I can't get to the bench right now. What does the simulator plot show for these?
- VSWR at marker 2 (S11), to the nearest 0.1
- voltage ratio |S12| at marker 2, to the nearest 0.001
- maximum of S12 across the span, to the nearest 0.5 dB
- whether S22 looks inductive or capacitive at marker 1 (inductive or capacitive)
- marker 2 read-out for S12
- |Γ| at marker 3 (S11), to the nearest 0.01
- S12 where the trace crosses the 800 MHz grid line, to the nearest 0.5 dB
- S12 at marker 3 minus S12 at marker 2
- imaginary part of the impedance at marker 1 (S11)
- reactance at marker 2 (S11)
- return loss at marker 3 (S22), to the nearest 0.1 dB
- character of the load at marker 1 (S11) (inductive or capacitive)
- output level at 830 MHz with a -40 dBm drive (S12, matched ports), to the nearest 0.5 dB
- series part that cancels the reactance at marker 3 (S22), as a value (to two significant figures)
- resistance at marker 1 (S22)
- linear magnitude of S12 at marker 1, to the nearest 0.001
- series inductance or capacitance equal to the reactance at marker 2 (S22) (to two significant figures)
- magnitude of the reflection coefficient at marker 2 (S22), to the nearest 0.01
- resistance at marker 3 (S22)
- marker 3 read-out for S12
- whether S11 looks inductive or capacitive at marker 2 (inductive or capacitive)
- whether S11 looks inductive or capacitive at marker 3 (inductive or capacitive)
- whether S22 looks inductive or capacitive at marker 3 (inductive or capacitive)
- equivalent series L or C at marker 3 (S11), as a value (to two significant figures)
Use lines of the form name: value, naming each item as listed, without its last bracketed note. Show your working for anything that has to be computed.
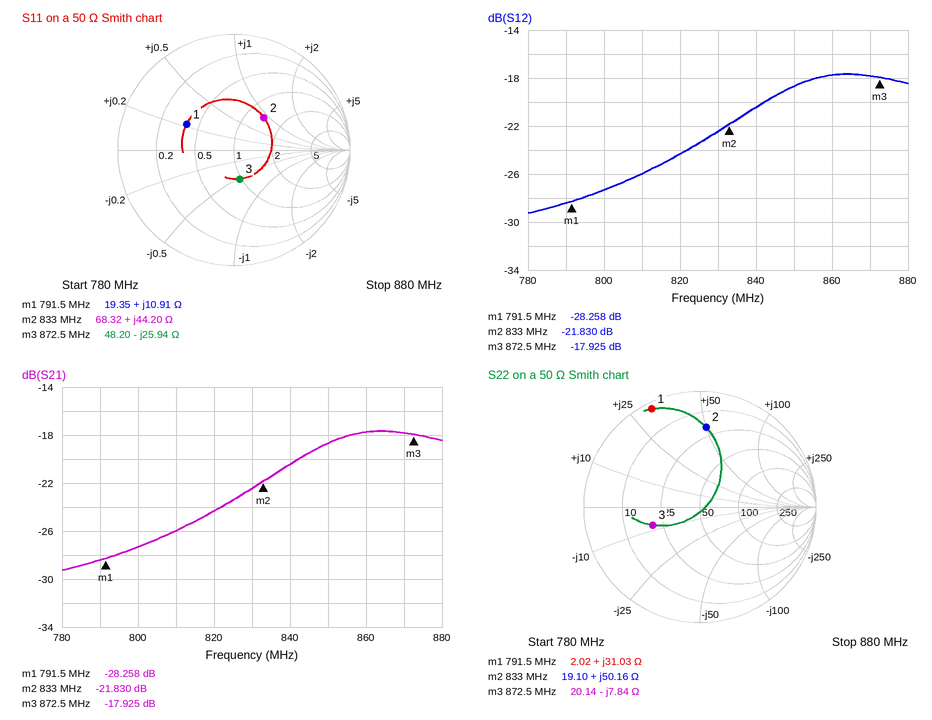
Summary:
VSWR at marker 2 (S11), to the nearest 0.1: 2.2
voltage ratio |S12| at marker 2, to the nearest 0.001: 10^(-21.83/20) ≈ 0.081
maximum of S12 across the span, to the nearest 0.5 dB: -17.5 dB
whether S22 looks inductive or capacitive at marker 1: inductive
marker 2 read-out for S12: -21.830 dB
|Γ| at marker 3 (S11), to the nearest 0.01: 0.26
S12 where the trace crosses the 800 MHz grid line, to the nearest 0.5 dB: -27.5 dB
S12 at marker 3 minus S12 at marker 2: -17.925 − (-21.83) = 3.905 dB
imaginary part of the impedance at marker 1: +10.91 Ω
reactance at marker 2: +44.20 Ω
return loss at marker 3 (S22), to the nearest 0.1 dB: 7.2 dB
character of the load at marker 1 (S11): inductive
output level at 830 MHz with a -40 dBm drive (S12, matched ports), to the nearest 0.5 dB: -40 dBm + (-22.5 dB) = -62.5 dBm
series part that cancels the reactance at marker 3 (S22), as a value: L = 7.84 Ω/(2π × 872.5 MHz) ≈ 1.4 nH
resistance at marker 1: 2.02 Ω
linear magnitude of S12 at marker 1, to the nearest 0.001: 10^(-28.258/20) ≈ 0.039
series inductance or capacitance equal to the reactance at marker 2 (S22): L = 50.16 Ω/(2π × 833 MHz) ≈ 9.6 nH
magnitude of the reflection coefficient at marker 2 (S22), to the nearest 0.01: 0.69
resistance at marker 3: 20.14 Ω
marker 3 read-out for S12: -17.925 dB
whether S11 looks inductive or capacitive at marker 2: inductive
whether S11 looks inductive or capacitive at marker 3: capacitive
whether S22 looks inductive or capacitive at marker 3: capacitive
equivalent series L or C at marker 3 (S11), as a value: C = 1/(2π × 872.5 MHz × 25.94 Ω) ≈ 7.0 pF
